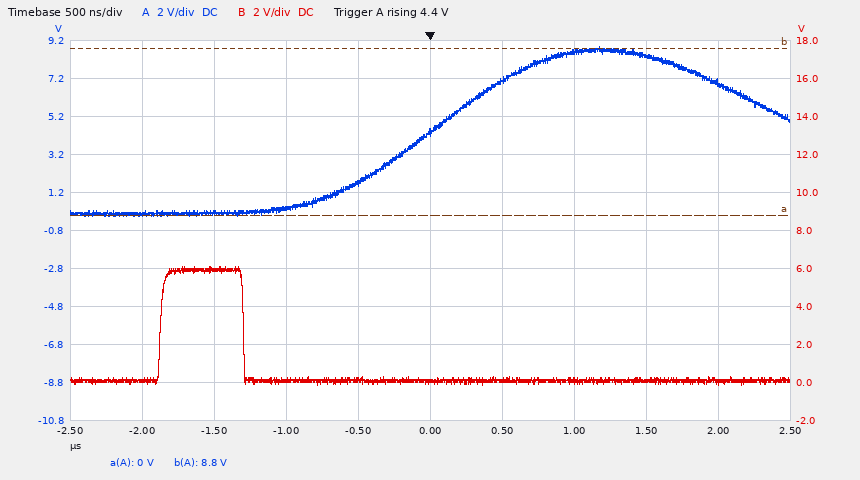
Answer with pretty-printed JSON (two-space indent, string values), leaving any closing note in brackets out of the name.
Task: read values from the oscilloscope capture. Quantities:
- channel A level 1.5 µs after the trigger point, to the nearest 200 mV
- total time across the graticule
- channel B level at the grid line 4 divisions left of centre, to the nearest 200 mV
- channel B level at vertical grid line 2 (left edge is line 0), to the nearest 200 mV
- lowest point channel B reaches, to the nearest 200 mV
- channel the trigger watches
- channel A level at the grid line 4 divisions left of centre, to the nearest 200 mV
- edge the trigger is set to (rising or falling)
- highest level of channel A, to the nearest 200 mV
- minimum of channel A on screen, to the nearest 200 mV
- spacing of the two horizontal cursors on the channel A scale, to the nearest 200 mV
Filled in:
{
  "channel A level 1.5 µs after the trigger point, to the nearest 200 mV": "8.4 V",
  "total time across the graticule": "5 µs",
  "channel B level at the grid line 4 divisions left of centre, to the nearest 200 mV": "200 mV",
  "channel B level at vertical grid line 2 (left edge is line 0), to the nearest 200 mV": "6.0 V",
  "lowest point channel B reaches, to the nearest 200 mV": "-200 mV",
  "channel the trigger watches": "channel A",
  "channel A level at the grid line 4 divisions left of centre, to the nearest 200 mV": "0.0 V",
  "edge the trigger is set to": "rising",
  "highest level of channel A, to the nearest 200 mV": "8.8 V",
  "minimum of channel A on screen, to the nearest 200 mV": "0.0 V",
  "spacing of the two horizontal cursors on the channel A scale, to the nearest 200 mV": "8.8 V"
}
